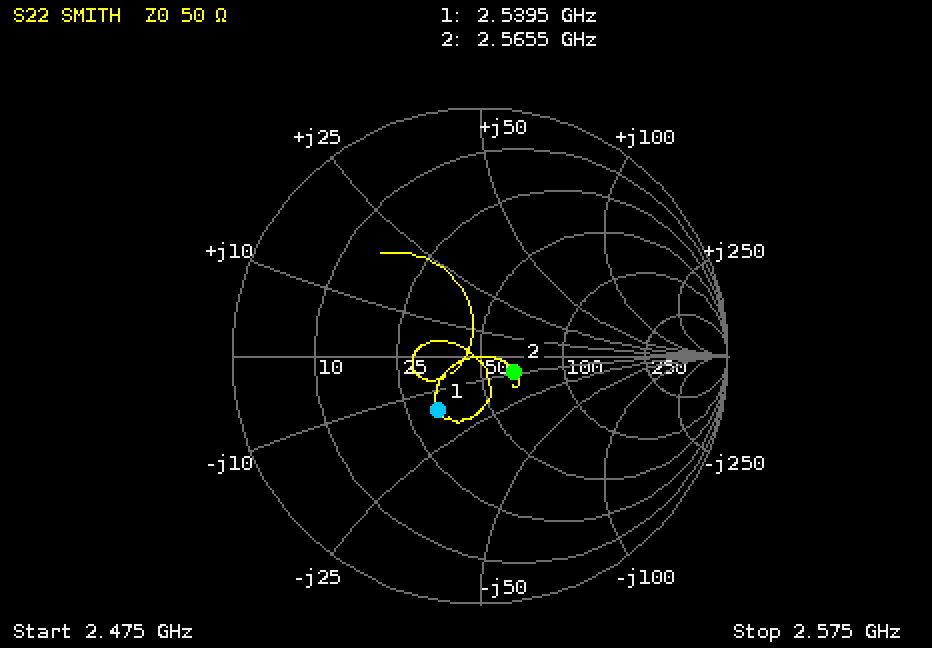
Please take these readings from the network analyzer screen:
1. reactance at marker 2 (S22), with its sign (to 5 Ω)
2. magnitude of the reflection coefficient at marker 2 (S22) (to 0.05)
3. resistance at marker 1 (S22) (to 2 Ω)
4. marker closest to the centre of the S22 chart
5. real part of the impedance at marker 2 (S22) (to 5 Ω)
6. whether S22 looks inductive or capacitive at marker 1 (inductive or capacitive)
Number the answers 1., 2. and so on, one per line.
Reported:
1. -10 Ω
2. 0.15
3. 32 Ω
4. marker 2
5. 65 Ω
6. capacitive
